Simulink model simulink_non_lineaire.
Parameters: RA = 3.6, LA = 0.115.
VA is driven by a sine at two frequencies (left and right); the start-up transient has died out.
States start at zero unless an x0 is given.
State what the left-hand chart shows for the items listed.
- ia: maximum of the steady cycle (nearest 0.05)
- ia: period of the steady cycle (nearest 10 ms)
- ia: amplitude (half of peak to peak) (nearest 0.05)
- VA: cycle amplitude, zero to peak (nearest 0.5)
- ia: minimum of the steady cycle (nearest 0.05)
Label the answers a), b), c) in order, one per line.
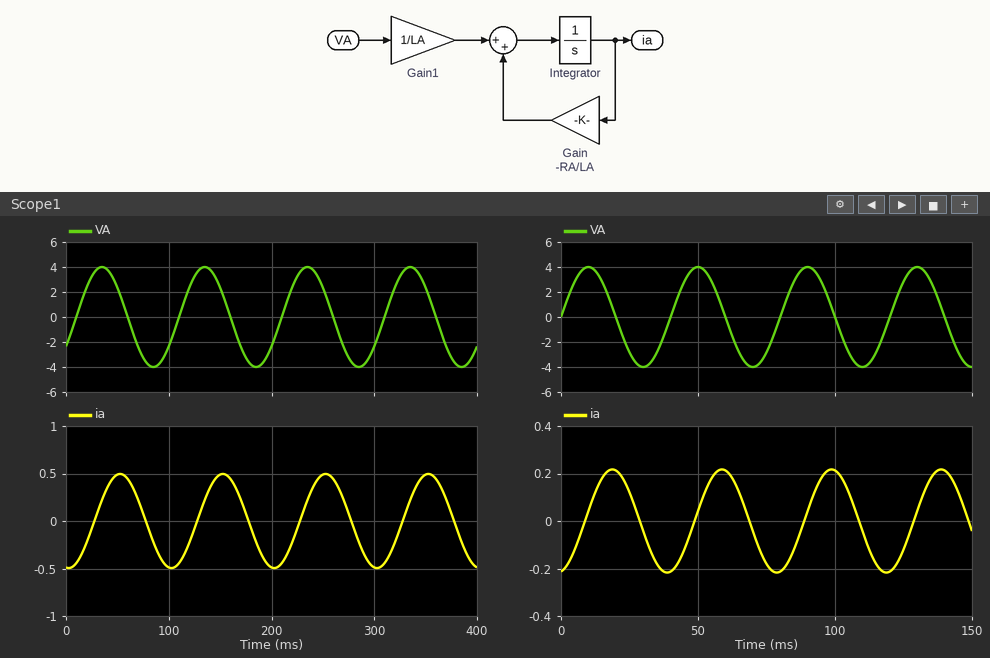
a) 0.50
b) 100 ms
c) 0.50
d) 4.0
e) -0.50
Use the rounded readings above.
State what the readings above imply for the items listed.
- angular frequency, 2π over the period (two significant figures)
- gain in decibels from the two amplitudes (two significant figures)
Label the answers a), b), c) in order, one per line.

a) 0.063 rad/ms
b) -18 dB
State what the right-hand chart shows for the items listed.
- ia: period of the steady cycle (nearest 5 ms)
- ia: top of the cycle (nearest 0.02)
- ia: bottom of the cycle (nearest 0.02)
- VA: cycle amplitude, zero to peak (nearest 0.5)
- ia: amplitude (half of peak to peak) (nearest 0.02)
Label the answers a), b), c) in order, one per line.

a) 40 ms
b) 0.22
c) -0.22
d) 4.0
e) 0.22
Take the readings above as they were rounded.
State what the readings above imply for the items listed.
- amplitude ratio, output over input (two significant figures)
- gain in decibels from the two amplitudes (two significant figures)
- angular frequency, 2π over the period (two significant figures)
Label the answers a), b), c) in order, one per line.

a) 0.055
b) -25 dB
c) 0.16 rad/ms
